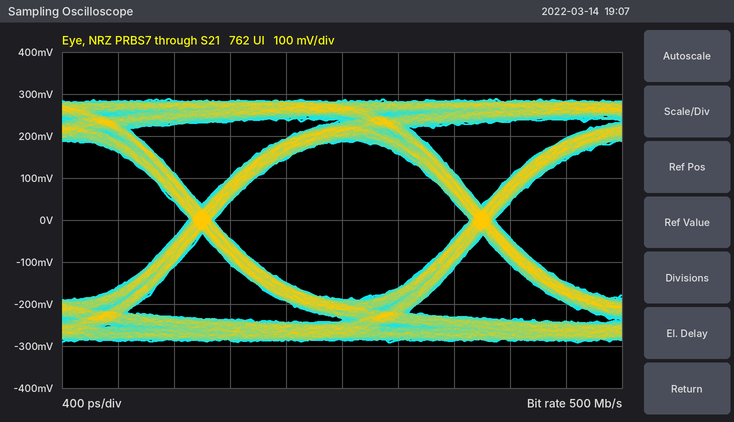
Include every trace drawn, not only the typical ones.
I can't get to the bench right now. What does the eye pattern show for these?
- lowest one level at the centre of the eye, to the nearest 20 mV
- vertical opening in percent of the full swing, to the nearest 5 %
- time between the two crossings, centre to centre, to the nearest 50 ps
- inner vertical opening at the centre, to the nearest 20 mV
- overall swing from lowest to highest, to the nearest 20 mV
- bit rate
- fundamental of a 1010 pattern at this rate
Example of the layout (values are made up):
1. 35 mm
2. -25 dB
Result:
1. 180 mV
2. 65 %
3. 2.00 ns
4. 380 mV
5. 580 mV
6. 500 Mb/s
7. 250 MHz
